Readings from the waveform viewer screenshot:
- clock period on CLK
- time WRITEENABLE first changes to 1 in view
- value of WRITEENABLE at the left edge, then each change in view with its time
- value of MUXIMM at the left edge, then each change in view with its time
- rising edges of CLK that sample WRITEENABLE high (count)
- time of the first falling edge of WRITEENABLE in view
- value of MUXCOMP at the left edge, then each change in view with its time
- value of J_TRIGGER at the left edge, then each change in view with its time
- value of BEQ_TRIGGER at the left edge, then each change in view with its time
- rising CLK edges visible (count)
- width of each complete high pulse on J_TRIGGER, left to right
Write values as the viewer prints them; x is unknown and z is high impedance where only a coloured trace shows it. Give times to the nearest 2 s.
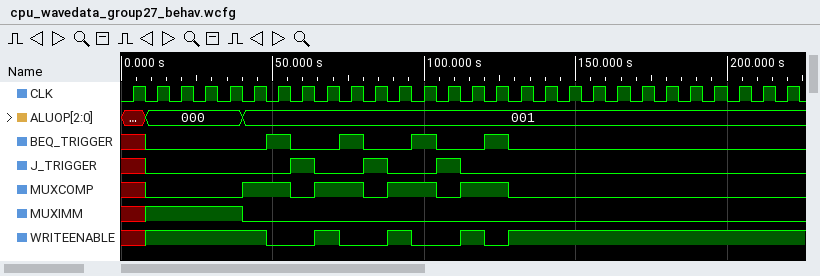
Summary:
8 s
8 s
x, 1 at 8 s, 0 at 48 s, 1 at 64 s, 0 at 72 s, 1 at 88 s, 0 at 96 s, 1 at 112 s, 0 at 120 s, 1 at 128 s
x, 1 at 8 s, 0 at 40 s
20
48 s
x, 0 at 8 s, 1 at 40 s, 0 at 56 s, 1 at 64 s, 0 at 80 s, 1 at 88 s, 0 at 104 s, 1 at 112 s, 0 at 128 s
x, 0 at 8 s, 1 at 56 s, 0 at 64 s, 1 at 80 s, 0 at 88 s, 1 at 104 s, 0 at 112 s
x, 0 at 8 s, 1 at 48 s, 0 at 56 s, 1 at 72 s, 0 at 80 s, 1 at 96 s, 0 at 104 s, 1 at 120 s, 0 at 128 s
28
8 s, 8 s, 8 s
